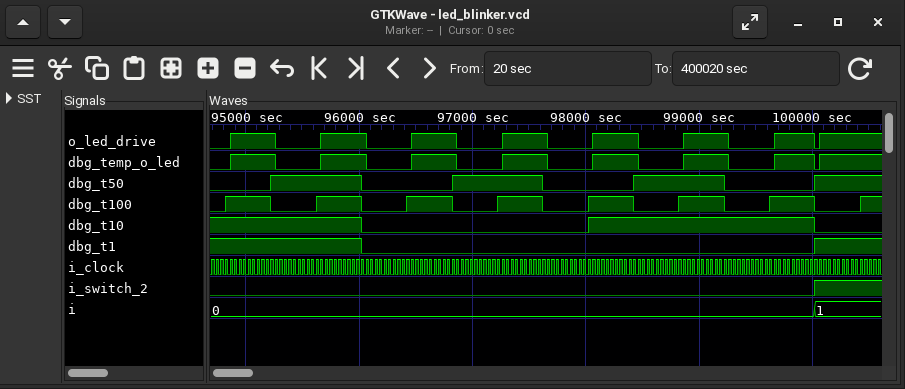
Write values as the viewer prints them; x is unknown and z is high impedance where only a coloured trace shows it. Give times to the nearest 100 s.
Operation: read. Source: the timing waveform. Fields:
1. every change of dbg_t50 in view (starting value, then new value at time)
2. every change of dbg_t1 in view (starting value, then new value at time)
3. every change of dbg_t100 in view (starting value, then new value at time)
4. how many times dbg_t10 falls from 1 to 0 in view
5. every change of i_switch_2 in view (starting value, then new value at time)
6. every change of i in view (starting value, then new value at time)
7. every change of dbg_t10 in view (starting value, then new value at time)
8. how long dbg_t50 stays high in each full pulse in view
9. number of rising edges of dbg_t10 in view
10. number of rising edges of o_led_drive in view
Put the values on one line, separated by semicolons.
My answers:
0, 1 at 95200 s, 0 at 96000 s, 1 at 96800 s, 0 at 97600 s, 1 at 98400 s, 0 at 99200 s, 1 at 100000 s; 1, 0 at 96000 s, 1 at 100000 s; 0, 1 at 94800 s, 0 at 95200 s, 1 at 95600 s, 0 at 96000 s, 1 at 96400 s, 0 at 96800 s, 1 at 97200 s, 0 at 97600 s, 1 at 98000 s, 0 at 98400 s, 1 at 98800 s, 0 at 99200 s, 1 at 99600 s, 0 at 100000 s, 1 at 100400 s; 2; 0, 1 at 100000 s; 0, 1 at 100000 s; 1, 0 at 96000 s, 1 at 98000 s, 0 at 100000 s; 800 s, 800 s, 800 s; 1; 8
